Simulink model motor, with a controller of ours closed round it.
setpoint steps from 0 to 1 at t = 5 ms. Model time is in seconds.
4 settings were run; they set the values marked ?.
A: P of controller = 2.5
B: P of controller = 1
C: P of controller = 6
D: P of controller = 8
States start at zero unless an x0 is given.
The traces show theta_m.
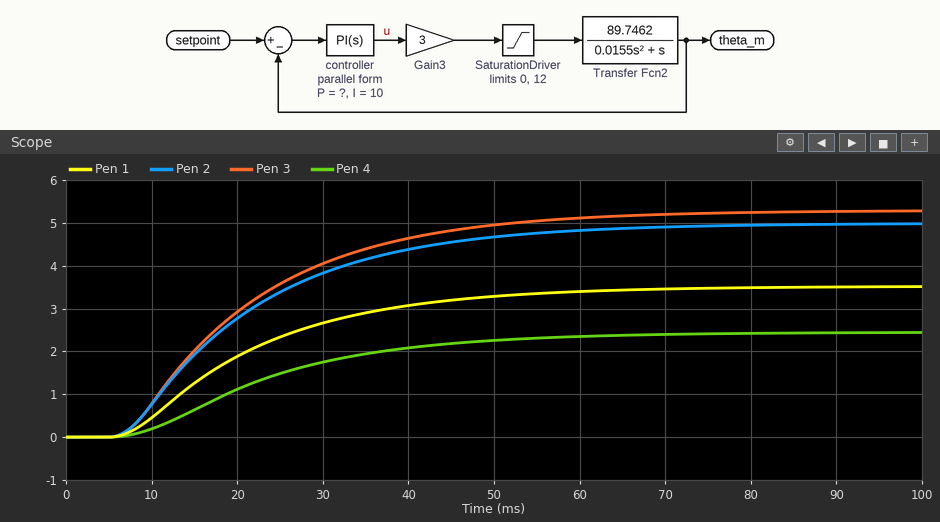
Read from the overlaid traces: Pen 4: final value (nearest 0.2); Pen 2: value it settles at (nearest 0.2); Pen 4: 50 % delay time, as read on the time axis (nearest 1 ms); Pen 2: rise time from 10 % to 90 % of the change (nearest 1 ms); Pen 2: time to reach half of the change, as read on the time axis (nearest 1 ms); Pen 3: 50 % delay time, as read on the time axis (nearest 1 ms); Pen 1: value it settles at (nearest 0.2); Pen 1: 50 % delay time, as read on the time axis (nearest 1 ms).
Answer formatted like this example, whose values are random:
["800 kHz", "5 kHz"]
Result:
["2.4", "5.0", "21 ms", "34 ms", "18 ms", "18 ms", "3.6", "19 ms"]
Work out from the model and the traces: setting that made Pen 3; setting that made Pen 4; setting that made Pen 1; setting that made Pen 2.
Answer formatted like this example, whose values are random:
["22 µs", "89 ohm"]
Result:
["D", "B", "A", "C"]
